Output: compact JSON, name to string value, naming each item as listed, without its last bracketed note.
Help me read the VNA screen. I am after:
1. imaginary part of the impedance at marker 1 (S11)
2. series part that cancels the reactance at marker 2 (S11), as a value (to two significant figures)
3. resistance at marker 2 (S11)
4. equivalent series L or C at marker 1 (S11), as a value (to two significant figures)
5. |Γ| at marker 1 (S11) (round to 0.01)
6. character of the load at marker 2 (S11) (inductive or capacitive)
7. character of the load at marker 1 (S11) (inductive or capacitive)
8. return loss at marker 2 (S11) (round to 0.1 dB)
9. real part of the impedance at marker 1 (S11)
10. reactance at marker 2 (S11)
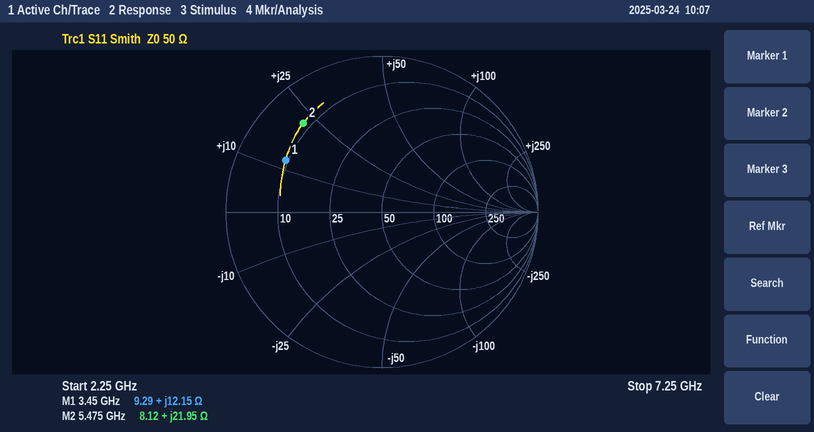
{"imaginary part of the impedance at marker 1": "+12.15 Ω", "series part that cancels the reactance at marker 2 (S11), as a value": "1.3 pF", "resistance at marker 2": "8.12 Ω", "equivalent series L or C at marker 1 (S11), as a value": "560 pH", "|Γ| at marker 1 (S11)": "0.70", "character of the load at marker 2 (S11)": "inductive", "character of the load at marker 1 (S11)": "inductive", "return loss at marker 2 (S11)": "2.4 dB", "real part of the impedance at marker 1": "9.29 Ω", "reactance at marker 2": "+21.95 Ω"}
